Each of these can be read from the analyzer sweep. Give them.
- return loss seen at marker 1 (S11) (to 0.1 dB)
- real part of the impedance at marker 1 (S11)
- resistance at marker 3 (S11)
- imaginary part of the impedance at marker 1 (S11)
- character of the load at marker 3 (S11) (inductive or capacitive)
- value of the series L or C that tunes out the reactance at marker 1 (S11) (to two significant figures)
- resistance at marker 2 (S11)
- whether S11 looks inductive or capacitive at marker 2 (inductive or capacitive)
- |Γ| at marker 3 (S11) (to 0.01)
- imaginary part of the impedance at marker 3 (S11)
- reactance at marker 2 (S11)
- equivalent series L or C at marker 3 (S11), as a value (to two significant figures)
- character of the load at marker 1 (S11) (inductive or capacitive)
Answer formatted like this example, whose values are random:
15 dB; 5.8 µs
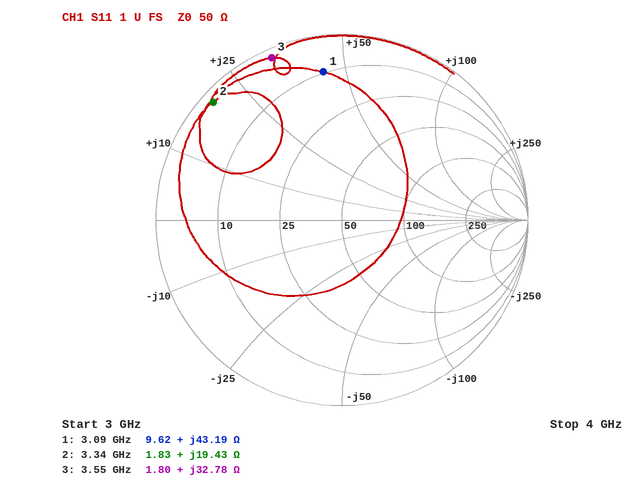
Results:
1.9 dB; 9.62 Ω; 1.80 Ω; +43.19 Ω; inductive; 1.2 pF; 1.83 Ω; inductive; 0.95; +32.78 Ω; +19.43 Ω; 1.5 nH; inductive
